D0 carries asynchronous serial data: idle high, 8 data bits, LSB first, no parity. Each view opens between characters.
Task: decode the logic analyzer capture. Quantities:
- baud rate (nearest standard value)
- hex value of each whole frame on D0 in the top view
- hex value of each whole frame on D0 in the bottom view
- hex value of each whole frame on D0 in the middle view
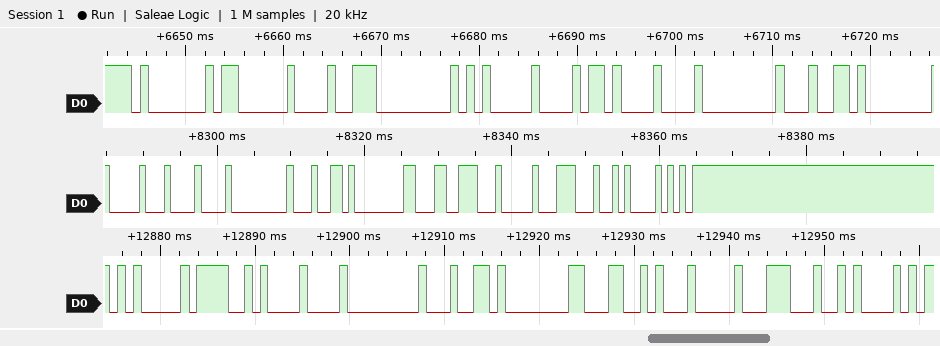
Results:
1200 baud
01, 03, C8, 00, 05, 68, 08, 00, 64
05, 4F, 08, 00, 64, 80, 4C, 04, 1C, 0A
10, 08, 00, 64, 80, CC, 04, 1C, 0A, F5
